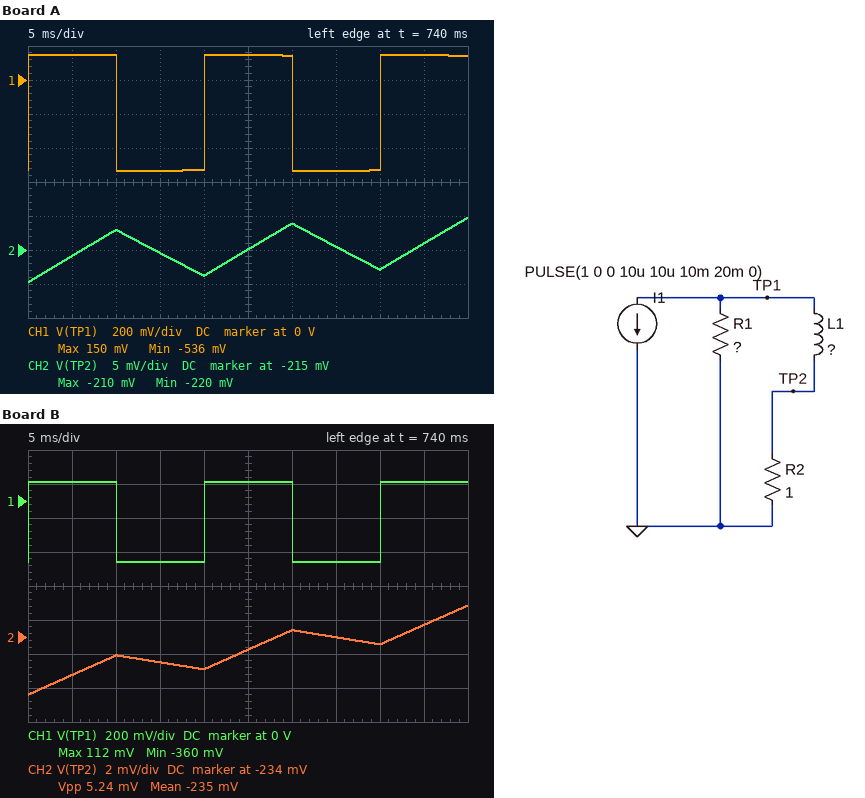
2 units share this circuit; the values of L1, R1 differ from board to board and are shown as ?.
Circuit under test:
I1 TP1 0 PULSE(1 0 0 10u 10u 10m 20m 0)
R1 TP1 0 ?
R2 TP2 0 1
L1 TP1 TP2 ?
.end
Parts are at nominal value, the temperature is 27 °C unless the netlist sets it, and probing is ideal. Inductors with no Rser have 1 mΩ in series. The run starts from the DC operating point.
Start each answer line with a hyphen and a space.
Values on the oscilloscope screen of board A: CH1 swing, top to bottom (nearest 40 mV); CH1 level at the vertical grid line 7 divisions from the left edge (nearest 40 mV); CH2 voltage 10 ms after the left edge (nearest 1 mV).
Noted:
- 680 mV
- -520 mV
- -212 mV
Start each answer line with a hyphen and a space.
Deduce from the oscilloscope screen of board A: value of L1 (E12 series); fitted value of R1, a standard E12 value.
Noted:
- 470 mH
- 0.68 Ω
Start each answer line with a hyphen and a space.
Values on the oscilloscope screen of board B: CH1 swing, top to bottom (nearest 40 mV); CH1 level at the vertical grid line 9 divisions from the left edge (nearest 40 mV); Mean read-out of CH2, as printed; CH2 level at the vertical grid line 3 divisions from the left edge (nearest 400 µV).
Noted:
- 480 mV
- 120 mV
- -235 mV
- -235.6 mV
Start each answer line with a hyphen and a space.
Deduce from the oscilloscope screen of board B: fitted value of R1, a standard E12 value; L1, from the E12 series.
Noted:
- 0.47 Ω
- 1.5 H
